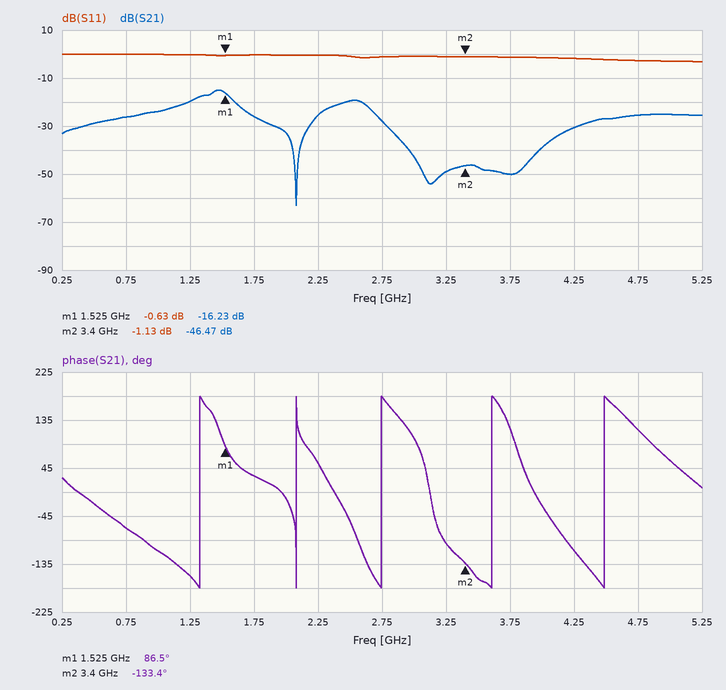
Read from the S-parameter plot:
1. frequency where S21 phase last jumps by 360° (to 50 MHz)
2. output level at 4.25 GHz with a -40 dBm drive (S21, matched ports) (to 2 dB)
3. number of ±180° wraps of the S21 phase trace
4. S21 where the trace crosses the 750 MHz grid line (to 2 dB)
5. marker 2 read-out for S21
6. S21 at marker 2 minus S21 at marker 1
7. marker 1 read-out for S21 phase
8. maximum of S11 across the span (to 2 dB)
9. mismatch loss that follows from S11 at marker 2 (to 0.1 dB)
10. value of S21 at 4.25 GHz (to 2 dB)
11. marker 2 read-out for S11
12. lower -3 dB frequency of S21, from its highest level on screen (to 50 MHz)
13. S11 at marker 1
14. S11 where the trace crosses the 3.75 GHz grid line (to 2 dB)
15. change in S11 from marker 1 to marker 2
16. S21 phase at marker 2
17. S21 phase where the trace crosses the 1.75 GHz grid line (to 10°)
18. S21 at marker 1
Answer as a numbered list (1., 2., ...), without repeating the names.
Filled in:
1. 4.50 GHz
2. -70 dBm
3. 5
4. -26 dB
5. -46.47 dB
6. -30.24 dB
7. 86.5°
8. 0 dB
9. 6.4 dB
10. -30 dB
11. -1.13 dB
12. 1.30 GHz
13. -0.63 dB
14. -2 dB
15. -0.50 dB
16. -133.4°
17. 30°
18. -16.23 dB
